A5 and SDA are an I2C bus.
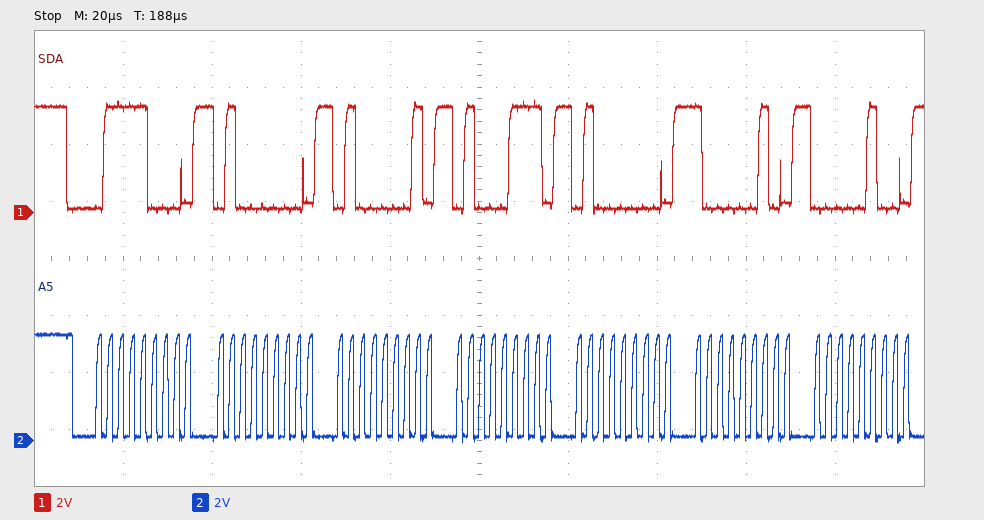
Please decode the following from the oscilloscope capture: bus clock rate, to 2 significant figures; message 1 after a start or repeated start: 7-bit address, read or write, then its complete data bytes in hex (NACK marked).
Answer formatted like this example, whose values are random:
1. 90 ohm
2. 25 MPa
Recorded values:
1. 400 kHz
2. 0x3C write: 40 41 47 40 82 04
